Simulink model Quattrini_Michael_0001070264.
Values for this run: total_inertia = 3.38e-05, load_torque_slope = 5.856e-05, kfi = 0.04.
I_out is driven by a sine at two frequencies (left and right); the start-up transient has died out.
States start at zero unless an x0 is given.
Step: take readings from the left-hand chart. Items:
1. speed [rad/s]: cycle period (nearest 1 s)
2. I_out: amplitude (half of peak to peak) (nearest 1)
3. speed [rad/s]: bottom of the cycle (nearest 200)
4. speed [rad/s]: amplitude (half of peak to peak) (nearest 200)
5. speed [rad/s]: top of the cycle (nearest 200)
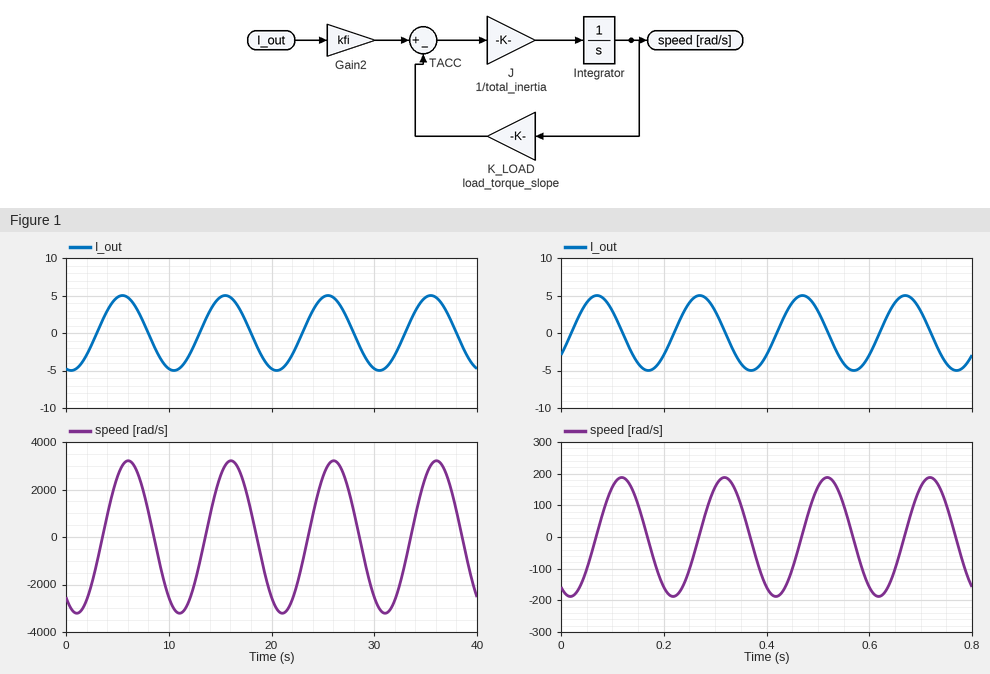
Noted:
10 s
5
-3200
3200
3200
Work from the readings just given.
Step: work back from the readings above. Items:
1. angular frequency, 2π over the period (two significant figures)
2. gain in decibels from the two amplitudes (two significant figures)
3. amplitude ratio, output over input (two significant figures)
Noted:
0.63 rad/s
56 dB
640
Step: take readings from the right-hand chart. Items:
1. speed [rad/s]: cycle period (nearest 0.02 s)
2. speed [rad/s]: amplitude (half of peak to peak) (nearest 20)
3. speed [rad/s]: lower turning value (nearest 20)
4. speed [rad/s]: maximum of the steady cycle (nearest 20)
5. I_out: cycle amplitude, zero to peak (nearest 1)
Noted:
0.20 s
180
-180
180
5
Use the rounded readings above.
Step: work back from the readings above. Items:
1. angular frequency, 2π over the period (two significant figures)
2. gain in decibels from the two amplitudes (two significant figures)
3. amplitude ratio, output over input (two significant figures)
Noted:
31 rad/s
31 dB
36
